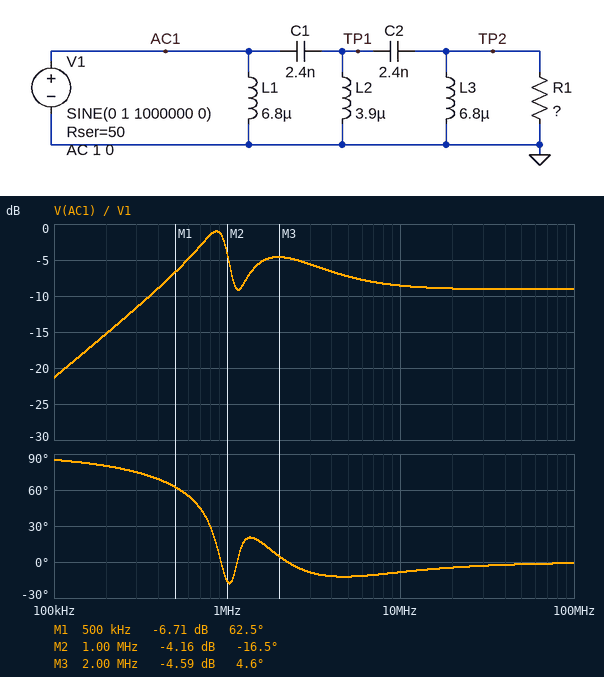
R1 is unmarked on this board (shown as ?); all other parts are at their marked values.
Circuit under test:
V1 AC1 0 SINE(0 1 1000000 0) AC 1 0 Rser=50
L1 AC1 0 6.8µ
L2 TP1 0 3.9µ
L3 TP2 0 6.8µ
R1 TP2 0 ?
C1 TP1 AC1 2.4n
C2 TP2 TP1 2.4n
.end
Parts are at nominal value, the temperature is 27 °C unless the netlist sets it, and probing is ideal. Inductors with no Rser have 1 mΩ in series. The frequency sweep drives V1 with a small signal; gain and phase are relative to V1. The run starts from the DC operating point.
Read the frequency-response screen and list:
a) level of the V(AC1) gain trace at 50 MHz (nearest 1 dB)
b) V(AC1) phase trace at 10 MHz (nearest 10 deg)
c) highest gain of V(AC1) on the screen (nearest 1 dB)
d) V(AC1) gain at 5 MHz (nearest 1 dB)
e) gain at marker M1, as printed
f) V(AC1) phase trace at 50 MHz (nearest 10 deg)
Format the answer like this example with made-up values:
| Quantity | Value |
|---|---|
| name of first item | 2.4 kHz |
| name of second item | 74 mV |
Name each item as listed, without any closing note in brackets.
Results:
| Quantity | Value |
|---|---|
| level of the V(AC1) gain trace at 50 MHz | -9 dB |
| V(AC1) phase trace at 10 MHz | -10 deg |
| highest gain of V(AC1) on the screen | -1 dB |
| V(AC1) gain at 5 MHz | -7 dB |
| gain at marker M1, as printed | -6.71 dB |
| V(AC1) phase trace at 50 MHz | 0 deg |
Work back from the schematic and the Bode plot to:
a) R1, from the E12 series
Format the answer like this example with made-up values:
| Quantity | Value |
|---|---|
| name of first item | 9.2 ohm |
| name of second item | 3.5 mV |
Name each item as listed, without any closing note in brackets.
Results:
| Quantity | Value |
|---|---|
| R1, from the E12 series | 27 Ω |
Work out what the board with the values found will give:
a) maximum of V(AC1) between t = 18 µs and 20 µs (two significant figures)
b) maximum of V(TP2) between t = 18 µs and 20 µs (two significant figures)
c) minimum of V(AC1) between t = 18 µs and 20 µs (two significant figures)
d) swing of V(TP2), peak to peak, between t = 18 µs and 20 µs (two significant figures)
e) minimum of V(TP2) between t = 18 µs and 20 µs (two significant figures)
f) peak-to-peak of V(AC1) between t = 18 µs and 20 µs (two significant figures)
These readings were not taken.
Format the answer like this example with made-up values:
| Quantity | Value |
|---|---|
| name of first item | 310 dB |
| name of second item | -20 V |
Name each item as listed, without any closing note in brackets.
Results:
| Quantity | Value |
|---|---|
| maximum of V(AC1) between t = 18 µs and 20 µs | 620 mV |
| maximum of V(TP2) between t = 18 µs and 20 µs | 340 mV |
| minimum of V(AC1) between t = 18 µs and 20 µs | -620 mV |
| swing of V(TP2), peak to peak, between t = 18 µs and 20 µs | 670 mV |
| minimum of V(TP2) between t = 18 µs and 20 µs | -340 mV |
| peak-to-peak of V(AC1) between t = 18 µs and 20 µs | 1.2 V |
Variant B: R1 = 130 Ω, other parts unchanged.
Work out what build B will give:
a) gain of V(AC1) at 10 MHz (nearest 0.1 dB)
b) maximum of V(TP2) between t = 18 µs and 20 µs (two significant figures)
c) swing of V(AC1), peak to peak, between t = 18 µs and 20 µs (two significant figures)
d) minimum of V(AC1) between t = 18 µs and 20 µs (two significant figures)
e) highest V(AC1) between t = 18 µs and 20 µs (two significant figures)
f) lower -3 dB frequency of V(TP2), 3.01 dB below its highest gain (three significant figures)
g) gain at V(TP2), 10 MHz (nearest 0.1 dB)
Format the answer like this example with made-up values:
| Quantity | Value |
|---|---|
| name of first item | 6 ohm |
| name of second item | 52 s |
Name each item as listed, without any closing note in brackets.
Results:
| Quantity | Value |
|---|---|
| gain of V(AC1) at 10 MHz | -3.4 dB |
| maximum of V(TP2) between t = 18 µs and 20 µs | 750 mV |
| swing of V(AC1), peak to peak, between t = 18 µs and 20 µs | 1.1 V |
| minimum of V(AC1) between t = 18 µs and 20 µs | -530 mV |
| highest V(AC1) between t = 18 µs and 20 µs | 530 mV |
| lower -3 dB frequency of V(TP2), 3.01 dB below its highest gain | 849 kHz |
| gain at V(TP2), 10 MHz | -3.0 dB |
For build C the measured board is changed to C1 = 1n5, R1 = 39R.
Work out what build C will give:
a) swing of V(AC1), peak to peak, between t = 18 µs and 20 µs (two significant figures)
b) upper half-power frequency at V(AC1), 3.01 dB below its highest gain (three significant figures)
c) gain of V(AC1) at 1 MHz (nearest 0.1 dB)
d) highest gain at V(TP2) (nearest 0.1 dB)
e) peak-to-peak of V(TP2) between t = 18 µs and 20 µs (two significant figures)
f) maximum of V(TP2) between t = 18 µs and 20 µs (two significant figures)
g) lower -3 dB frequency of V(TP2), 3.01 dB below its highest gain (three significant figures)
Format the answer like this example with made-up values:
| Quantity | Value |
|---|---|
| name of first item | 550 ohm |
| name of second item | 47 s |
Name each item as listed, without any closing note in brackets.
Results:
| Quantity | Value |
|---|---|
| swing of V(AC1), peak to peak, between t = 18 µs and 20 µs | 1.6 V |
| upper half-power frequency at V(AC1), 3.01 dB below its highest gain | 2.40 MHz |
| gain of V(AC1) at 1 MHz | -1.8 dB |
| highest gain at V(TP2) | -7.2 dB |
| peak-to-peak of V(TP2) between t = 18 µs and 20 µs | 540 mV |
| maximum of V(TP2) between t = 18 µs and 20 µs | 270 mV |
| lower -3 dB frequency of V(TP2), 3.01 dB below its highest gain | 1.03 MHz |
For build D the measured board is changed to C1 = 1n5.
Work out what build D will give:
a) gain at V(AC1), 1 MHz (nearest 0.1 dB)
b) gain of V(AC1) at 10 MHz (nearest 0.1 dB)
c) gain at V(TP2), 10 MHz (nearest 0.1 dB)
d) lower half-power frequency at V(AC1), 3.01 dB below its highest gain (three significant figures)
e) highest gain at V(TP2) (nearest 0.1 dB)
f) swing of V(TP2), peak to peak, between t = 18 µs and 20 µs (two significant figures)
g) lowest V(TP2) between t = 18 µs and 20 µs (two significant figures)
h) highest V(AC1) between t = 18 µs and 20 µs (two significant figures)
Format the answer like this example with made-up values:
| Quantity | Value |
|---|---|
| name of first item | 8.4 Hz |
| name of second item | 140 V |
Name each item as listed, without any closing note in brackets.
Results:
| Quantity | Value |
|---|---|
| gain at V(AC1), 1 MHz | -1.5 dB |
| gain of V(AC1) at 10 MHz | -8.2 dB |
| gain at V(TP2), 10 MHz | -9.1 dB |
| lower half-power frequency at V(AC1), 3.01 dB below its highest gain | 682 kHz |
| highest gain at V(TP2) | -8.9 dB |
| swing of V(TP2), peak to peak, between t = 18 µs and 20 µs | 390 mV |
| lowest V(TP2) between t = 18 µs and 20 µs | -200 mV |
| highest V(AC1) between t = 18 µs and 20 µs | 840 mV |
